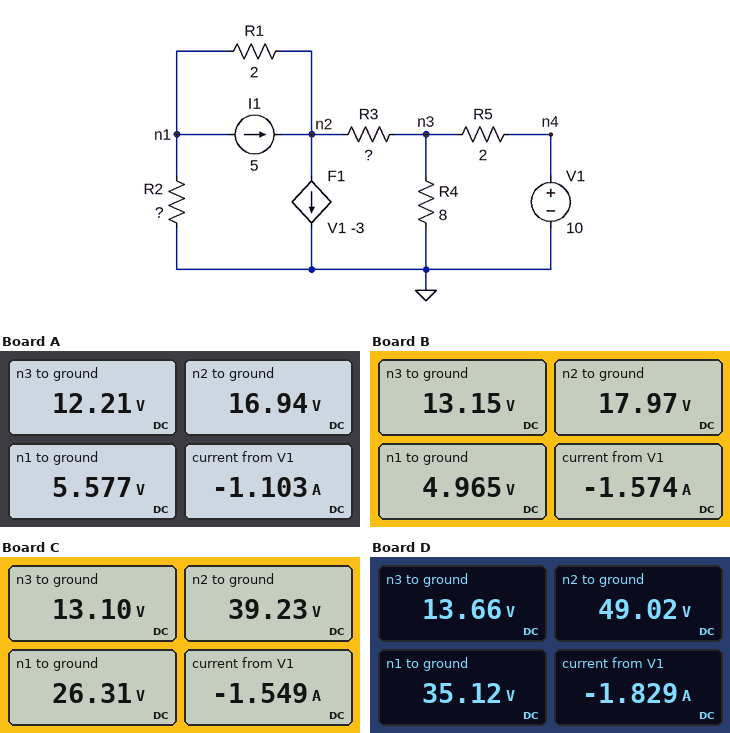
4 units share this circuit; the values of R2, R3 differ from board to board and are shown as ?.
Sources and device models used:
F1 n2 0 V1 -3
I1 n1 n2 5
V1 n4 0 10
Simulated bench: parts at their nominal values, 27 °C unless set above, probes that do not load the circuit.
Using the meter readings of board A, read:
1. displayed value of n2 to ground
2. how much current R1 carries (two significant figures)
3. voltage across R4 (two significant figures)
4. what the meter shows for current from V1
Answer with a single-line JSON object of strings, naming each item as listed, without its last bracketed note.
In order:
{"displayed value of n2 to ground": "16.94 V", "how much current R1 carries": "5.7 A", "voltage across R4": "12 V", "what the meter shows for current from V1": "-1.103 A"}
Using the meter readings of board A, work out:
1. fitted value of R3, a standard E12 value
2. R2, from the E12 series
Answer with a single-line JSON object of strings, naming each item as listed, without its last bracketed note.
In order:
{"fitted value of R3, a standard E12 value": "1.8 Ω", "R2, from the E12 series": "8.2 Ω"}
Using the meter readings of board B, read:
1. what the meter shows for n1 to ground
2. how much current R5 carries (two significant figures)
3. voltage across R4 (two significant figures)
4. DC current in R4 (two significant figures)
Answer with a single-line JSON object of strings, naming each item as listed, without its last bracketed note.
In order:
{"what the meter shows for n1 to ground": "4.965 V", "how much current R5 carries": "1.6 A", "voltage across R4": "13 V", "DC current in R4": "1.6 A"}
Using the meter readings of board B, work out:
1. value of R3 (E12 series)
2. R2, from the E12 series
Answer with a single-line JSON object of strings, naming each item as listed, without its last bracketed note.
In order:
{"value of R3": "1.5 Ω", "R2, from the E12 series": "3.3 Ω"}
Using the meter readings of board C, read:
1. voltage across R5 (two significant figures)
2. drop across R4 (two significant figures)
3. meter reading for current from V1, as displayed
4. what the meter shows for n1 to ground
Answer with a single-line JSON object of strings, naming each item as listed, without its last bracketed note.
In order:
{"voltage across R5": "3.1 V", "drop across R4": "13 V", "meter reading for current from V1, as displayed": "-1.549 A", "what the meter shows for n1 to ground": "26.31 V"}
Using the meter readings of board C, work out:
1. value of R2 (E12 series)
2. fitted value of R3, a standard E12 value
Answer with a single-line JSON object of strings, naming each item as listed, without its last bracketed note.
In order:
{"value of R2": "18 Ω", "fitted value of R3, a standard E12 value": "8.2 Ω"}
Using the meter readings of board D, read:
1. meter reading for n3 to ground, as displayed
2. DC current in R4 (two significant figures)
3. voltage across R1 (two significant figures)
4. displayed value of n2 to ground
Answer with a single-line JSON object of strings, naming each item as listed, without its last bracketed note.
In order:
{"meter reading for n3 to ground, as displayed": "13.66 V", "DC current in R4": "1.7 A", "voltage across R1": "14 V", "displayed value of n2 to ground": "49.02 V"}
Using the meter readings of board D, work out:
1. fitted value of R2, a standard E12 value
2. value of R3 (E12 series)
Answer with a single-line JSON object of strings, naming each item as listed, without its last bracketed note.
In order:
{"fitted value of R2, a standard E12 value": "18 Ω", "value of R3": "10 Ω"}
